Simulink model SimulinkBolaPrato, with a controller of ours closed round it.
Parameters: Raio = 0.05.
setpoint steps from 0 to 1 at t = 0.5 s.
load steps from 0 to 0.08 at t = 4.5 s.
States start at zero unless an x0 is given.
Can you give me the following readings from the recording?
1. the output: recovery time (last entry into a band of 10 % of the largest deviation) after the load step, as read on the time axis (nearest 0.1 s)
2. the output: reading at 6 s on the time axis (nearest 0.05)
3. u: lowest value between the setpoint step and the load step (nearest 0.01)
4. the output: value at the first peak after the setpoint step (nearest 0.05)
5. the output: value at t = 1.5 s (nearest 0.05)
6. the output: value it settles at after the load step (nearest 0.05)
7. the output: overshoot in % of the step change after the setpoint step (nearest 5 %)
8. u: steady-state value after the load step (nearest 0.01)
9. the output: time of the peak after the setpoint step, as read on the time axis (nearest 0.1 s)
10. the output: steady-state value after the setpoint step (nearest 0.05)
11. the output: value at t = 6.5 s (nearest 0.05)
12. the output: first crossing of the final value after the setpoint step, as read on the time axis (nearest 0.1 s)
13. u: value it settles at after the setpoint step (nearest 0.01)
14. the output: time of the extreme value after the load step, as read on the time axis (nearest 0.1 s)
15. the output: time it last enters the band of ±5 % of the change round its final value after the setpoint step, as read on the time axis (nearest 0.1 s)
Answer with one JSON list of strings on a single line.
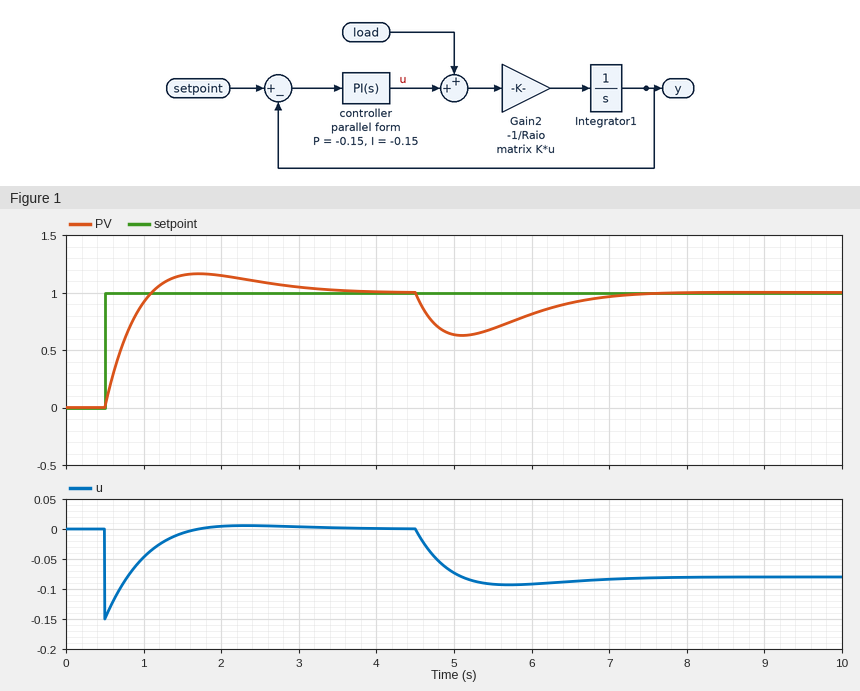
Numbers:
["7.0 s", "0.80", "-0.15", "1.15", "1.15", "1.00", "15 %", "-0.08", "1.7 s", "1.00", "0.90", "1.1 s", "0.00", "5.1 s", "3.0 s"]
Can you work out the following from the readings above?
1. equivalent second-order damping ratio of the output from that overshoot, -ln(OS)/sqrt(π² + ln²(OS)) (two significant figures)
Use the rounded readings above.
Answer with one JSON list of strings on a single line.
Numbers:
["0.52"]
